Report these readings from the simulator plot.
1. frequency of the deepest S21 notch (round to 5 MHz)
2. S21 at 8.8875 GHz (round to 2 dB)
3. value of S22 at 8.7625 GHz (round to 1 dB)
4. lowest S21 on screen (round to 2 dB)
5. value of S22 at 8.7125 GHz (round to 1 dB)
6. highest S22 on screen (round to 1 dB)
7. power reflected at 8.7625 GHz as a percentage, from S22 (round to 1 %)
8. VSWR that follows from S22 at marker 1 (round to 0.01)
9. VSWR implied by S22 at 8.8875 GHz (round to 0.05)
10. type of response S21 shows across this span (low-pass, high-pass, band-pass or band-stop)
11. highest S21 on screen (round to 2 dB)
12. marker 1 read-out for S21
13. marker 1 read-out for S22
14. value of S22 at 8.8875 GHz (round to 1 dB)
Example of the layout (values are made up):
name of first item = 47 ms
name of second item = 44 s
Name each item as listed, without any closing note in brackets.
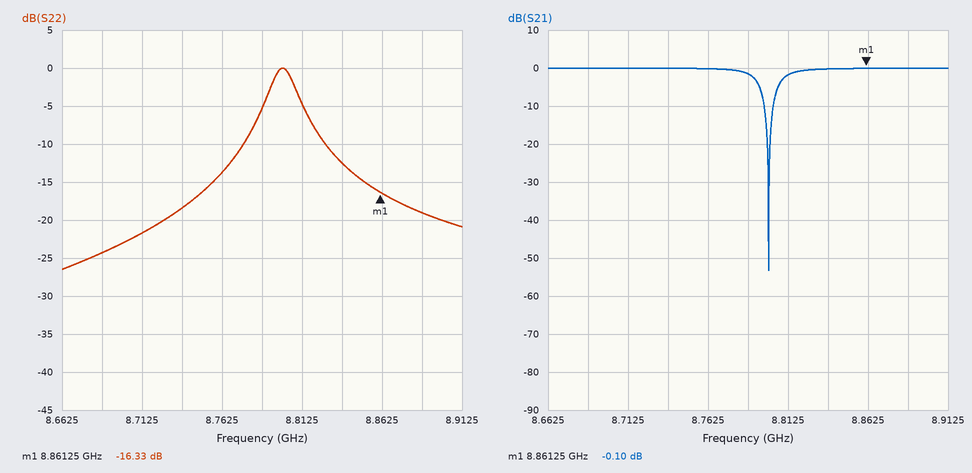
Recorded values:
frequency of the deepest S21 notch = 8.800 GHz
S21 at 8.8875 GHz = 0 dB
value of S22 at 8.7625 GHz = -14 dB
lowest S21 on screen = -54 dB
value of S22 at 8.7125 GHz = -22 dB
highest S22 on screen = 0 dB
power reflected at 8.7625 GHz as a percentage, from S22 = 4 %
VSWR that follows from S22 at marker 1 = 1.36
VSWR implied by S22 at 8.8875 GHz = 1.25
type of response S21 shows across this span = band-stop
highest S21 on screen = 0 dB
marker 1 read-out for S21 = -0.10 dB
marker 1 read-out for S22 = -16.33 dB
value of S22 at 8.8875 GHz = -19 dB
